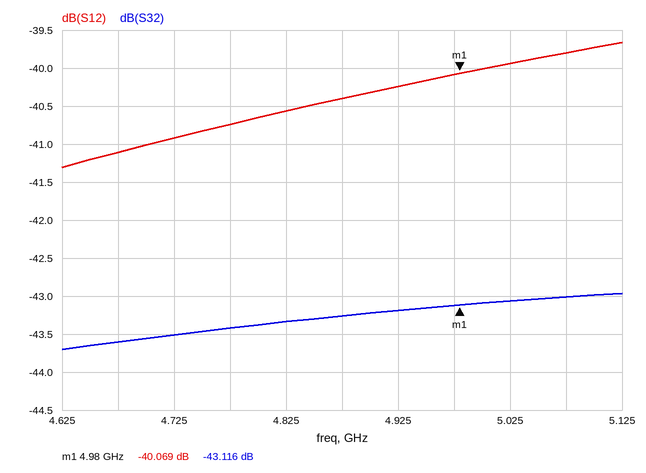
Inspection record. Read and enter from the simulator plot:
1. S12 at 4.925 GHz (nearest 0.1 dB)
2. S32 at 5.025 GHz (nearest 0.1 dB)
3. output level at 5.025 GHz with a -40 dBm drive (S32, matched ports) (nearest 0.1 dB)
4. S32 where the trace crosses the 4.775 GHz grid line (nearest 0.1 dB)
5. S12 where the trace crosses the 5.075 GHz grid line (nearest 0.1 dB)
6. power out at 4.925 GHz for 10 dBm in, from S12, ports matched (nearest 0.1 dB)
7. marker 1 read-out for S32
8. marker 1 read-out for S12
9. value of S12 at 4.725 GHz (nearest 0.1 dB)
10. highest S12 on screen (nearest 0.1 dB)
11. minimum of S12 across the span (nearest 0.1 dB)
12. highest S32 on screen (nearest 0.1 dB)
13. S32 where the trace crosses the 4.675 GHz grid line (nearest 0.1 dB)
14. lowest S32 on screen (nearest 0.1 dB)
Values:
-40.2 dB
-43.1 dB
-83.1 dBm
-43.4 dB
-39.8 dB
-30.2 dBm
-43.116 dB
-40.069 dB
-40.9 dB
-39.7 dB
-41.3 dB
-43.0 dB
-43.6 dB
-43.7 dB
